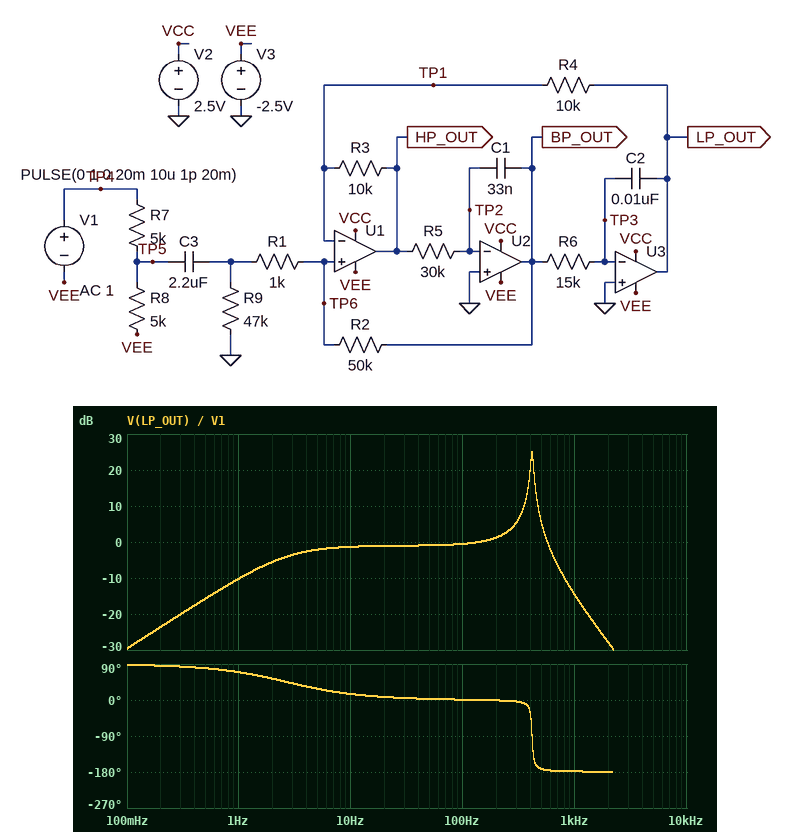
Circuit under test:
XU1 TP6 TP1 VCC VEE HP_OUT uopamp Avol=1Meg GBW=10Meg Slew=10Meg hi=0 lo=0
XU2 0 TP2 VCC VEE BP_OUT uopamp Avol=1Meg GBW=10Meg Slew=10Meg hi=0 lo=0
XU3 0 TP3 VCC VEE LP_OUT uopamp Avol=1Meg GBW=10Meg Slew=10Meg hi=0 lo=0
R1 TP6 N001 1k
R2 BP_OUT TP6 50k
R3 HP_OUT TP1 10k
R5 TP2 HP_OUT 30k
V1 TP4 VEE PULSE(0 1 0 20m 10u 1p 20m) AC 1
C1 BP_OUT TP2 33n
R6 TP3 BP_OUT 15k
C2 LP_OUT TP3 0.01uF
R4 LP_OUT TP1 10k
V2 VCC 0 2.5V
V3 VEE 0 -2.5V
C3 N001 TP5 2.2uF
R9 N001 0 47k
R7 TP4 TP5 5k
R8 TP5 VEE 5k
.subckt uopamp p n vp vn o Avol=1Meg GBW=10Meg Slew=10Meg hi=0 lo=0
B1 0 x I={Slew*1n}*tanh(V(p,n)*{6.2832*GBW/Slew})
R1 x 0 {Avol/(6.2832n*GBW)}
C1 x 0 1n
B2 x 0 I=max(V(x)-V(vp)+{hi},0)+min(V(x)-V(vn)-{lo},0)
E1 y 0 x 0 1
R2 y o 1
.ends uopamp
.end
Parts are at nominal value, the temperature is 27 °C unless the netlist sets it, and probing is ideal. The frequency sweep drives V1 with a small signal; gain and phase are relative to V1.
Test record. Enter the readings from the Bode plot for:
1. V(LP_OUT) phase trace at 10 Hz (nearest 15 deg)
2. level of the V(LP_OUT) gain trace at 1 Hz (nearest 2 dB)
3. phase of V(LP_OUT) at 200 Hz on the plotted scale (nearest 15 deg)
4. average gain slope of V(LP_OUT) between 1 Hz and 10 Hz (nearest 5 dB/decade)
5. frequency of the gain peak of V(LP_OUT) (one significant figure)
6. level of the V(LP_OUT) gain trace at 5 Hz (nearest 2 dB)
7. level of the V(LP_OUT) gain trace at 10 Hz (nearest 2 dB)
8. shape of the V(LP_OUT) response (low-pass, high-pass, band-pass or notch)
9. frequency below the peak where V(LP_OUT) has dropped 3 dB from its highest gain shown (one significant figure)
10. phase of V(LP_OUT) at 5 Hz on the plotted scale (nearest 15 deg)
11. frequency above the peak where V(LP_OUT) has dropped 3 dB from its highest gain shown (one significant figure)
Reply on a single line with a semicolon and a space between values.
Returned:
15 deg; -10 dB; 0 deg; 10 dB/decade; 400 Hz; -2 dB; -2 dB; band-pass; 400 Hz; 30 deg; 400 Hz
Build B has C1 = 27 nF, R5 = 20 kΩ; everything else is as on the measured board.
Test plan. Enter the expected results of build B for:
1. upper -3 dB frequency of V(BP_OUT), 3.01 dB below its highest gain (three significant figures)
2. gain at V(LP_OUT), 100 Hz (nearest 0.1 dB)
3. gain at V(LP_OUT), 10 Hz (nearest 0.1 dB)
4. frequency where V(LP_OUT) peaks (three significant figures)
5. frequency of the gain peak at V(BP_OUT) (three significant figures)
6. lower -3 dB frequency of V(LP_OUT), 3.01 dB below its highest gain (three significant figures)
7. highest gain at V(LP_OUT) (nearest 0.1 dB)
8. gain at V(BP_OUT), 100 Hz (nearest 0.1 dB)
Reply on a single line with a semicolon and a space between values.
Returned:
579 Hz; -0.8 dB; -1.3 dB; 559 Hz; 560 Hz; 540 Hz; 22.5 dB; -21.3 dB
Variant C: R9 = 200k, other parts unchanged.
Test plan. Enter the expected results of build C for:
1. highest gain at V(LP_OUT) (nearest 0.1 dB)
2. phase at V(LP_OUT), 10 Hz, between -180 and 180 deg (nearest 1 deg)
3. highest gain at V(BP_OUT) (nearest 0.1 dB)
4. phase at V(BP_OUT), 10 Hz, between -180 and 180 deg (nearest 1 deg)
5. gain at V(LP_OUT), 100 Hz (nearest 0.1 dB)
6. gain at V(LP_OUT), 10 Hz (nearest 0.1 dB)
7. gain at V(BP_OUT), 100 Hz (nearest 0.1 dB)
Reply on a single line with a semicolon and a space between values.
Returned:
25.3 dB; 9 deg; 17.1 dB; -81 deg; -0.2 dB; -0.8 dB; -20.7 dB
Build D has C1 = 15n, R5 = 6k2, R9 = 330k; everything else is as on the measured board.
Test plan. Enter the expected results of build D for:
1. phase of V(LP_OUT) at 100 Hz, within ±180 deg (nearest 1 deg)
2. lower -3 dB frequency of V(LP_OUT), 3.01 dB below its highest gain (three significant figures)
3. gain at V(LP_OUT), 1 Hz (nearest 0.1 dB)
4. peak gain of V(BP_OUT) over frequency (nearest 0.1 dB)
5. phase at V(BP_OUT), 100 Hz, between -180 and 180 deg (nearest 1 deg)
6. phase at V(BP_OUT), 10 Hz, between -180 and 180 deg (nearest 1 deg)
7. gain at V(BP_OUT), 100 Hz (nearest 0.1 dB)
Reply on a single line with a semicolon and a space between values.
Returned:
0 deg; 1.22 kHz; -6.0 dB; 17.1 dB; -90 deg; -81 deg; -21.1 dB
